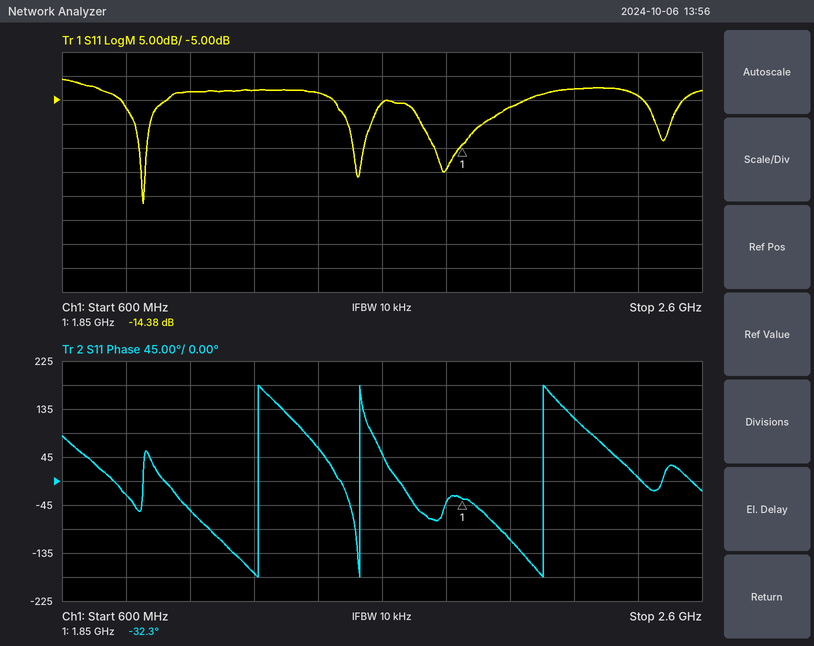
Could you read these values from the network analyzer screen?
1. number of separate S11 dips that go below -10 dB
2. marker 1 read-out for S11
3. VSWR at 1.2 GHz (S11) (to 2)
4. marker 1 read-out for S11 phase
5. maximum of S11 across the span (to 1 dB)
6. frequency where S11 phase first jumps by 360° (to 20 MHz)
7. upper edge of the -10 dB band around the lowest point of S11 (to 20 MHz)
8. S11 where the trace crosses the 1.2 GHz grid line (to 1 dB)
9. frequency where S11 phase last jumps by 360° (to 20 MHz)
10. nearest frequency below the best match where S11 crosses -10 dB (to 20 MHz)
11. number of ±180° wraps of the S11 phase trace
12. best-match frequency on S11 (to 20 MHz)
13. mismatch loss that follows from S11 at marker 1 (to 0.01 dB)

4
-14.38 dB
6
-32.3°
-1 dB
1.22 GHz
880 MHz
-3 dB
2.10 GHz
820 MHz
3
860 MHz
0.16 dB
